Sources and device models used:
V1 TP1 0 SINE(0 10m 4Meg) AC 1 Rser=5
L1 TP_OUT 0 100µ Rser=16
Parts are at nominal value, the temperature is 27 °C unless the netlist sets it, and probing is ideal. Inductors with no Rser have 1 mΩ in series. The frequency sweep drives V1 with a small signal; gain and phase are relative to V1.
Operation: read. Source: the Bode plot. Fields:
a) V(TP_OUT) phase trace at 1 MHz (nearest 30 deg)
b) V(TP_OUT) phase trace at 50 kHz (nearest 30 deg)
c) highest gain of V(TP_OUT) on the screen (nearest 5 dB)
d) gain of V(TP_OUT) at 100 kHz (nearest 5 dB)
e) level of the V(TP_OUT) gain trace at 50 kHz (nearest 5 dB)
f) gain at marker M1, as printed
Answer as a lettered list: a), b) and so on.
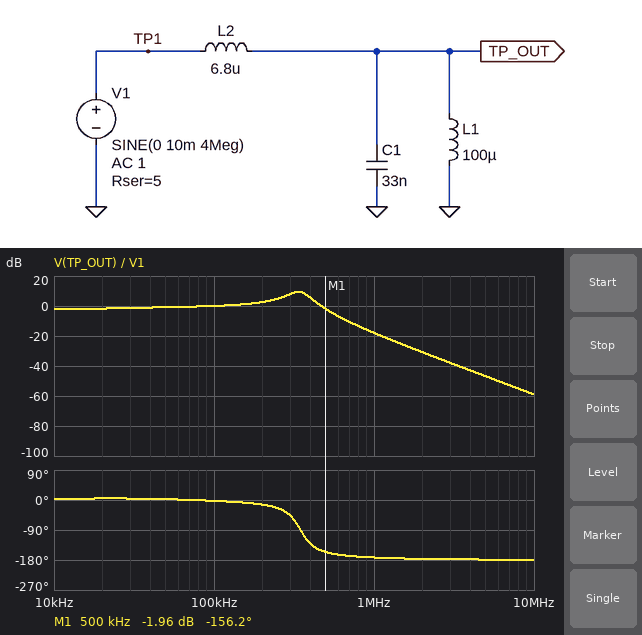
a) -180 deg
b) 0 deg
c) 10 dB
d) 0 dB
e) 0 dB
f) -1.96 dB
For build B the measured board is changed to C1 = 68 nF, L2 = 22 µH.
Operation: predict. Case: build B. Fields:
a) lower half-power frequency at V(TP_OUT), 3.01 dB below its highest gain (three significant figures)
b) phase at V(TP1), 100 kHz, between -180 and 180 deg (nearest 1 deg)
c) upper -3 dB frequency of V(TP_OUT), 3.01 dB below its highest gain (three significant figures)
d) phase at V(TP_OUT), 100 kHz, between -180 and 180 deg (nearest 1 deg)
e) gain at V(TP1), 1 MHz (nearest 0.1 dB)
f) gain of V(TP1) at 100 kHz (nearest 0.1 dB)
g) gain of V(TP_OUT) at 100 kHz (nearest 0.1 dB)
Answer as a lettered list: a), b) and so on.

a) 123 kHz
b) -12 deg
c) 158 kHz
d) -17 deg
e) 0 dB
f) -0.6 dB
g) 3.6 dB
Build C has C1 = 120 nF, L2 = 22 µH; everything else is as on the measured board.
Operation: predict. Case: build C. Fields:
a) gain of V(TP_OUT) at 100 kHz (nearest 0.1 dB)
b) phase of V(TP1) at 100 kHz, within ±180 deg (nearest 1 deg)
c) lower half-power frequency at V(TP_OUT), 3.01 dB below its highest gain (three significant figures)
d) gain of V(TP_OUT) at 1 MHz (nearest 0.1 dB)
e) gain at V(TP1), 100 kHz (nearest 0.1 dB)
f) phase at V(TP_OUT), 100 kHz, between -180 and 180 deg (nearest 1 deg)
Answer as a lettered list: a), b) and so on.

a) 8.0 dB
b) -45 deg
c) 86.4 kHz
d) -40.3 dB
e) -7.3 dB
f) -63 deg
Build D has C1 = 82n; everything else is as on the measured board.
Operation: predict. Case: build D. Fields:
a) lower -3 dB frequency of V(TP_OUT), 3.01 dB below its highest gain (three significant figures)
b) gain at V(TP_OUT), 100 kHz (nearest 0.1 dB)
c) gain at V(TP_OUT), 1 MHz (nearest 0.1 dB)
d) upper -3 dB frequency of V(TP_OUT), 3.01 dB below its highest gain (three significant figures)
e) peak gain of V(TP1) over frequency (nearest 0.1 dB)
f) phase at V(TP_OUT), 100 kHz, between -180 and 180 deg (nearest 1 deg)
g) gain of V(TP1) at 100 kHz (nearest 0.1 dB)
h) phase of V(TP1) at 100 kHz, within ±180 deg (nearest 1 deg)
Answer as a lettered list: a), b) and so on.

a) 136 kHz
b) 1.1 dB
c) -26.5 dB
d) 256 kHz
e) 0 dB
f) -13 deg
g) -0.4 dB
h) -12 deg
